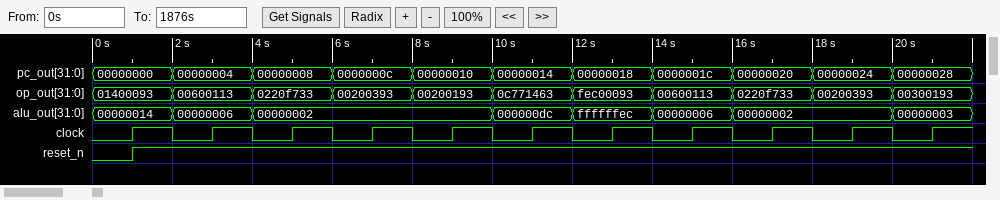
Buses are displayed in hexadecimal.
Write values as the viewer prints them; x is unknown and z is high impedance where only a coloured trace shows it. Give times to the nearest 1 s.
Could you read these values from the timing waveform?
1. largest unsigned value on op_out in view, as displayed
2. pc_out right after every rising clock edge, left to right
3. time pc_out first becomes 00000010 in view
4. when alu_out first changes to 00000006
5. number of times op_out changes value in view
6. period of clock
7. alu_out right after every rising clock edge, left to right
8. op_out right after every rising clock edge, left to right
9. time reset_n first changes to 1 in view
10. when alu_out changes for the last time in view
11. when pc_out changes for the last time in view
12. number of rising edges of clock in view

fec00093
00000000, 00000004, 00000008, 0000000c, 00000010, 00000014, 00000018, 0000001c, 00000020, 00000024, 00000028
8 s
2 s
10
2 s
00000014, 00000006, 00000002, 00000002, 00000002, 000000dc, ffffffec, 00000006, 00000002, 00000002, 00000003
01400093, 00600113, 0220f733, 00200393, 00200193, 0c771463, fec00093, 00600113, 0220f733, 00200393, 00300193
1 s
20 s
20 s
11
